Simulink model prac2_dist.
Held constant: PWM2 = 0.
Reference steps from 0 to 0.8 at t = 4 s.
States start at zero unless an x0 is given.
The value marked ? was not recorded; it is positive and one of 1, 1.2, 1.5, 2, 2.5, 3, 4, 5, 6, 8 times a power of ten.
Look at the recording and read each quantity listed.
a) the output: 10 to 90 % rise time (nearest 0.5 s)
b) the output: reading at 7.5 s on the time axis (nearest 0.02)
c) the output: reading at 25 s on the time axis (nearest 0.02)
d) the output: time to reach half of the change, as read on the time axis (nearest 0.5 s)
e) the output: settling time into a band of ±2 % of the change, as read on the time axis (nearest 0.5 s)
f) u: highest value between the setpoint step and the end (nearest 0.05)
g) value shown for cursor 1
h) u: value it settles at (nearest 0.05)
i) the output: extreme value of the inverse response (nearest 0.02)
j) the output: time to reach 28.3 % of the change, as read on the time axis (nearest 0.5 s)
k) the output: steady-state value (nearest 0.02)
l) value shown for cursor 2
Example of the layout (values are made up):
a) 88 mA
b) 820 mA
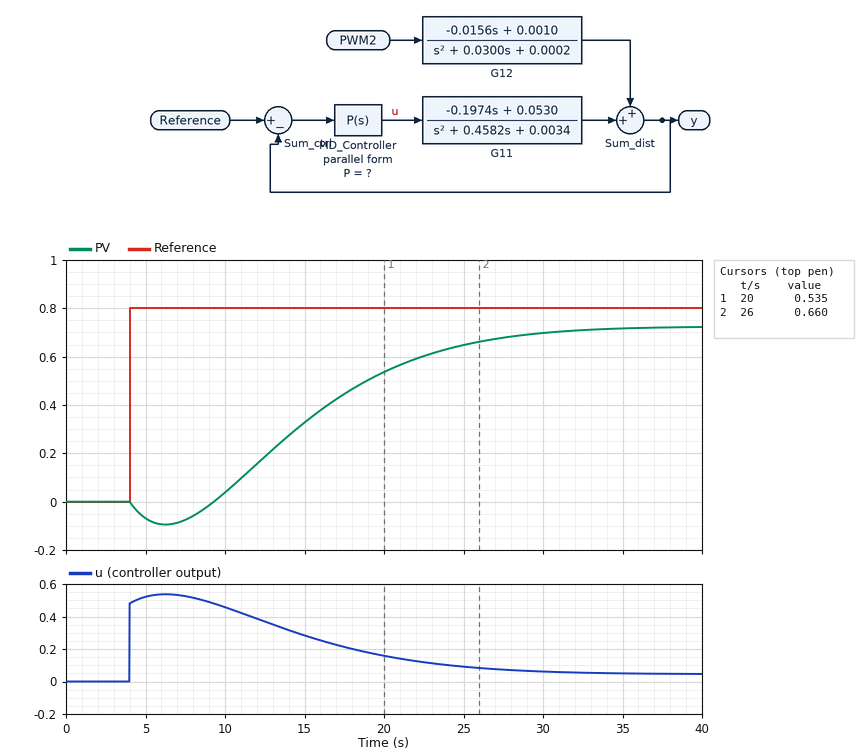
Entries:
a) 14.5 s
b) -0.08
c) 0.64
d) 15.5 s
e) 32.0 s
f) 0.55
g) 0.535
h) 0.05
i) -0.10
j) 13.0 s
k) 0.72
l) 0.660
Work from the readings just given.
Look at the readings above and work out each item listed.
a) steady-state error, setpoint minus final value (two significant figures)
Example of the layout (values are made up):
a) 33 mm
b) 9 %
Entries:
a) 0.080
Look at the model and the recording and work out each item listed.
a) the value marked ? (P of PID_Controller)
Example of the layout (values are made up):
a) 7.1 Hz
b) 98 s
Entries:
a) 0.6
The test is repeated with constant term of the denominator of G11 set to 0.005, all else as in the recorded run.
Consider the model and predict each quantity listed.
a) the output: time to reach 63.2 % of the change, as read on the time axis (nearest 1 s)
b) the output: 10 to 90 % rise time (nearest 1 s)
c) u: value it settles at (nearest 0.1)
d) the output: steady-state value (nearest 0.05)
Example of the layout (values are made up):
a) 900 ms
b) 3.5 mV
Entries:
a) 17 s
b) 14 s
c) 0.1
d) 0.70
